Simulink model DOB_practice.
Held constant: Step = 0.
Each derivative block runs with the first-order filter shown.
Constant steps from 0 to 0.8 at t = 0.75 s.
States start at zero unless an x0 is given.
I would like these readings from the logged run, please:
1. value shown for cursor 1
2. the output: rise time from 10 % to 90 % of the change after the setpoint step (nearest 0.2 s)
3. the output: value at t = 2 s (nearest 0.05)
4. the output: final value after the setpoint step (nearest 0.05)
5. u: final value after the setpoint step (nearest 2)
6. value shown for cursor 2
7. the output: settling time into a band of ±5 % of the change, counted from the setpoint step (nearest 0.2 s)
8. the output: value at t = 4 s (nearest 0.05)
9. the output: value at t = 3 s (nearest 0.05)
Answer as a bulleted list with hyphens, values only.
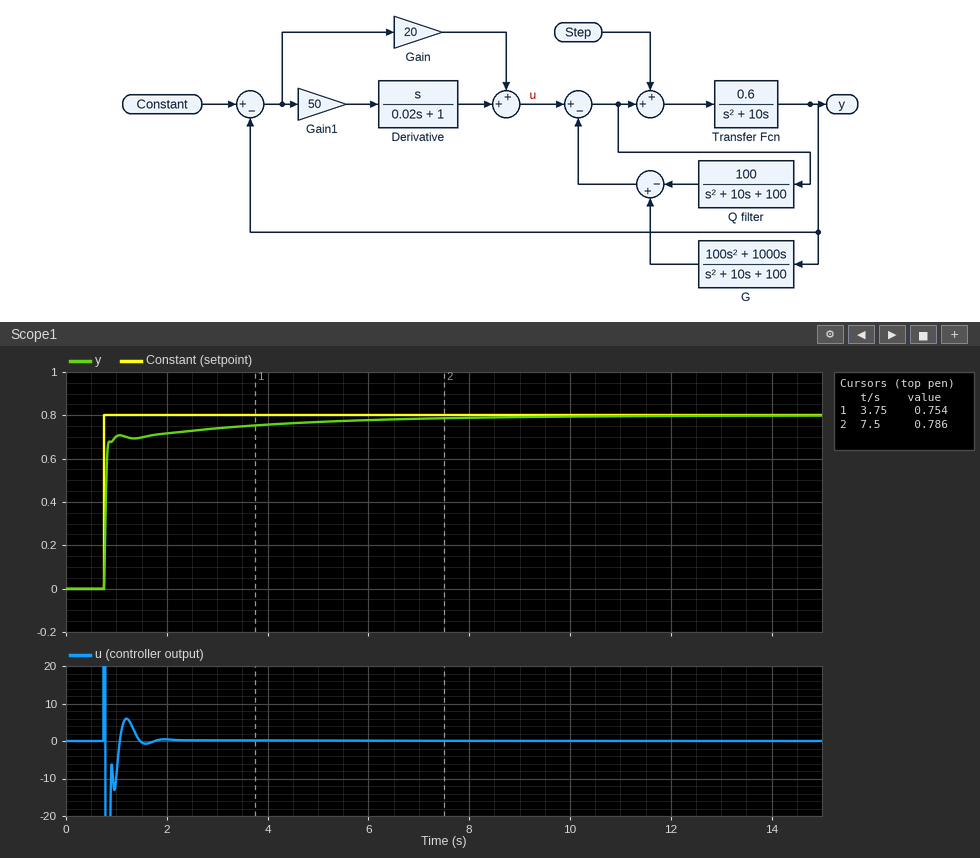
- 0.754
- 1.4 s
- 0.70
- 0.80
- 0
- 0.786
- 3.4 s
- 0.75
- 0.75
